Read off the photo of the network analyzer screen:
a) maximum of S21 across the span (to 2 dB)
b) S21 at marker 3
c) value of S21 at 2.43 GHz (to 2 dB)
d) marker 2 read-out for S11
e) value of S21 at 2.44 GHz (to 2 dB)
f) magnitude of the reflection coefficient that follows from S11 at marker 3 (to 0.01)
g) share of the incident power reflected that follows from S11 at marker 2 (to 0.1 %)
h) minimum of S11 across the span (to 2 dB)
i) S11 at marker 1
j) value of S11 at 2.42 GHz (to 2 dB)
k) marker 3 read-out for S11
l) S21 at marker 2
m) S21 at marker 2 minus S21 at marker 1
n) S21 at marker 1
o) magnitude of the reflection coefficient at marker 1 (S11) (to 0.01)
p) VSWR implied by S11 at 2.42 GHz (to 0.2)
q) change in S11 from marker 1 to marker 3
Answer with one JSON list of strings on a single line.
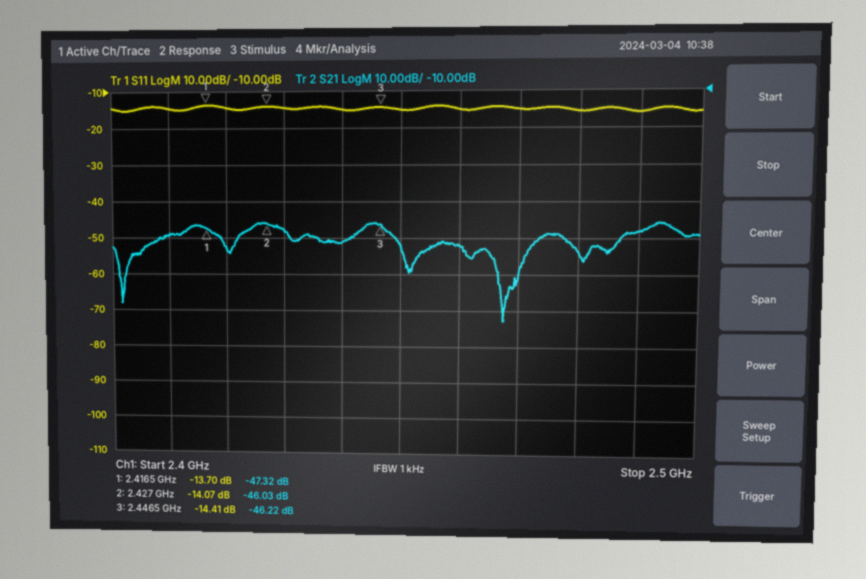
["-46 dB", "-46.22 dB", "-48 dB", "-14.07 dB", "-52 dB", "0.19", "3.9 %", "-16 dB", "-13.70 dB", "-14 dB", "-14.41 dB", "-46.03 dB", "1.29 dB", "-47.32 dB", "0.21", "1.4", "-0.71 dB"]
